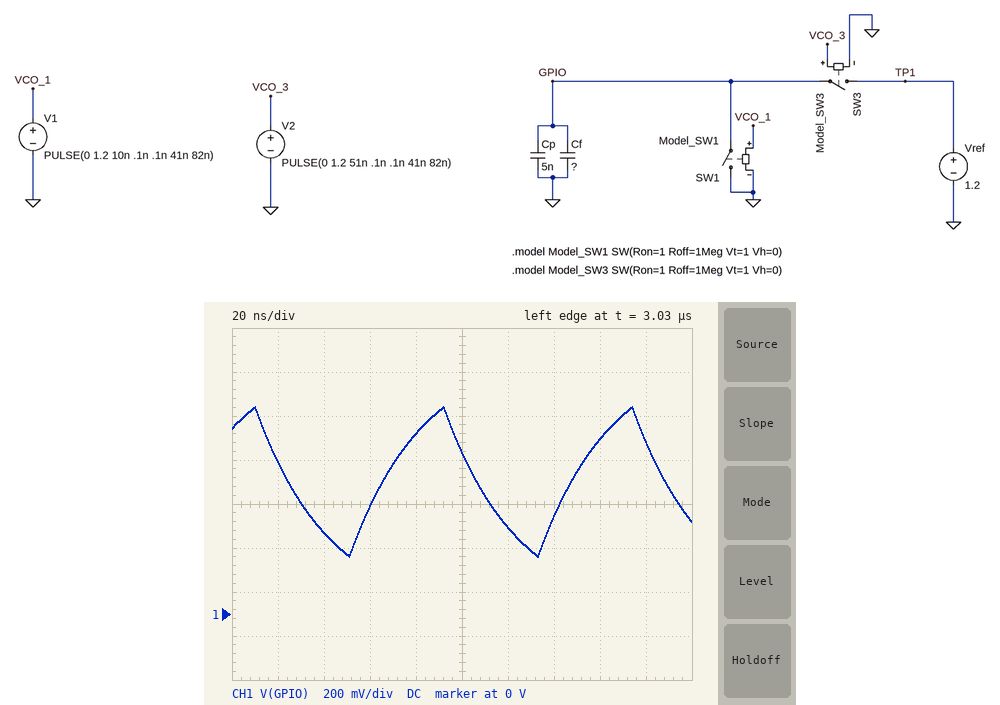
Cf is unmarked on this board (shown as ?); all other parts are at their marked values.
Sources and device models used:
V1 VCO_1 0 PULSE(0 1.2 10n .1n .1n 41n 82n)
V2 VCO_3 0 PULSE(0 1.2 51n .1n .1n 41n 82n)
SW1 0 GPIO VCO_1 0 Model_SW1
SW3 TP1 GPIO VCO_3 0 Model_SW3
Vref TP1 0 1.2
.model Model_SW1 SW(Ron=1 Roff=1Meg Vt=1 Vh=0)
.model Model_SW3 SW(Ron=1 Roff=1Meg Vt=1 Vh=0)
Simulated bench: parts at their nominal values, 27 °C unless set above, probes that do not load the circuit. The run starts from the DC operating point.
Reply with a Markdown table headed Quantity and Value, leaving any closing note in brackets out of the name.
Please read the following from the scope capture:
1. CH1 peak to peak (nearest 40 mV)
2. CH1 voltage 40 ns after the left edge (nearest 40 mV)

| Quantity | Value |
|---|---|
| CH1 peak to peak | 680 mV |
| CH1 voltage 40 ns after the left edge | 360 mV |
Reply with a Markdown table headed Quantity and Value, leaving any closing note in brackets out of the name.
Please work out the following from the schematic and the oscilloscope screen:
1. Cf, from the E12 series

| Quantity | Value |
|---|---|
| Cf, from the E12 series | 27 nF |
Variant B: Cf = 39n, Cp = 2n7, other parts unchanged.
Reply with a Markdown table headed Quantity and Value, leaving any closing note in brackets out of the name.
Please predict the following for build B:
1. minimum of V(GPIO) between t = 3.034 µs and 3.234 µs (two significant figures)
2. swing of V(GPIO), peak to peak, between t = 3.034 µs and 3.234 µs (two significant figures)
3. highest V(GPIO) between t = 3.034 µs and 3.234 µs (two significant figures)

| Quantity | Value |
|---|---|
| minimum of V(GPIO) between t = 3.034 µs and 3.234 µs | 330 mV |
| swing of V(GPIO), peak to peak, between t = 3.034 µs and 3.234 µs | 550 mV |
| highest V(GPIO) between t = 3.034 µs and 3.234 µs | 870 mV |
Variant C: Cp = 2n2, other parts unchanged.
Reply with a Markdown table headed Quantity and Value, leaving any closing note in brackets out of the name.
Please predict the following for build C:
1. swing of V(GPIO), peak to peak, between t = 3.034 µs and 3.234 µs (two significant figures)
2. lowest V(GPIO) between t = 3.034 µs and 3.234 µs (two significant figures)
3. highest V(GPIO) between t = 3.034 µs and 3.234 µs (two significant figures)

| Quantity | Value |
|---|---|
| swing of V(GPIO), peak to peak, between t = 3.034 µs and 3.234 µs | 730 mV |
| lowest V(GPIO) between t = 3.034 µs and 3.234 µs | 240 mV |
| highest V(GPIO) between t = 3.034 µs and 3.234 µs | 960 mV |
